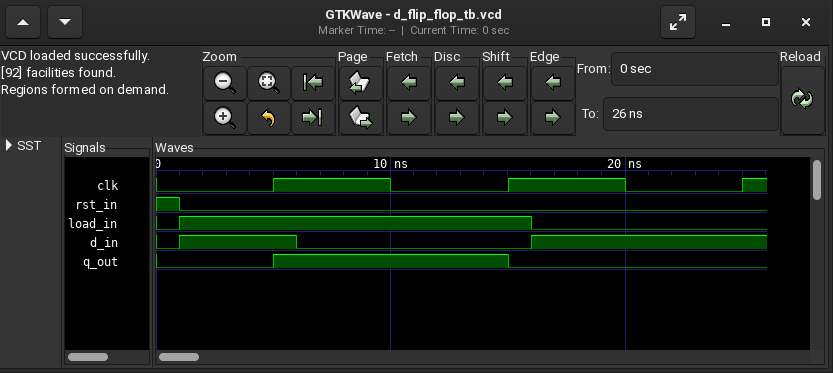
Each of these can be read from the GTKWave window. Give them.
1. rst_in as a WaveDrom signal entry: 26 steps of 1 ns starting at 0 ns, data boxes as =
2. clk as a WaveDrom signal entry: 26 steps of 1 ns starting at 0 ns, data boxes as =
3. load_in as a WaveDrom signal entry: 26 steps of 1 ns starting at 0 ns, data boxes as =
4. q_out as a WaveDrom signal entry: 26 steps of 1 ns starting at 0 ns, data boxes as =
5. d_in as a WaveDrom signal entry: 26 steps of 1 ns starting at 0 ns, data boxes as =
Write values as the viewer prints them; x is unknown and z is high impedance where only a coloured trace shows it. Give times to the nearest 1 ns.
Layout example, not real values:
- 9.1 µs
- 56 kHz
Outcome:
- {name: 'rst_in', wave: '10........................'}
- {name: 'clk', wave: '0....1....0....1....0....1'}
- {name: 'load_in', wave: '01..............0.........'}
- {name: 'q_out', wave: '0....1.........0..........'}
- {name: 'd_in', wave: '01....0.........1.........'}
